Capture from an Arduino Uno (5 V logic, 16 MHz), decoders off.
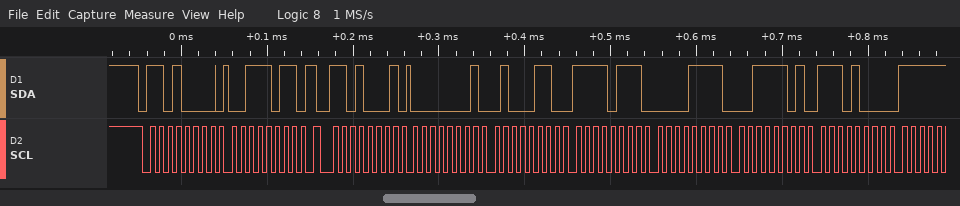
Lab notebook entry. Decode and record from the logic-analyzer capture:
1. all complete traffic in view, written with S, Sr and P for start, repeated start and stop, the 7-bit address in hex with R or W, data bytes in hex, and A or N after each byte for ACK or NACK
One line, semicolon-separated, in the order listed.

S 68W A 3B A Sr 68R A 01 A 46 A F7 A 0F A 3D A E8 A
